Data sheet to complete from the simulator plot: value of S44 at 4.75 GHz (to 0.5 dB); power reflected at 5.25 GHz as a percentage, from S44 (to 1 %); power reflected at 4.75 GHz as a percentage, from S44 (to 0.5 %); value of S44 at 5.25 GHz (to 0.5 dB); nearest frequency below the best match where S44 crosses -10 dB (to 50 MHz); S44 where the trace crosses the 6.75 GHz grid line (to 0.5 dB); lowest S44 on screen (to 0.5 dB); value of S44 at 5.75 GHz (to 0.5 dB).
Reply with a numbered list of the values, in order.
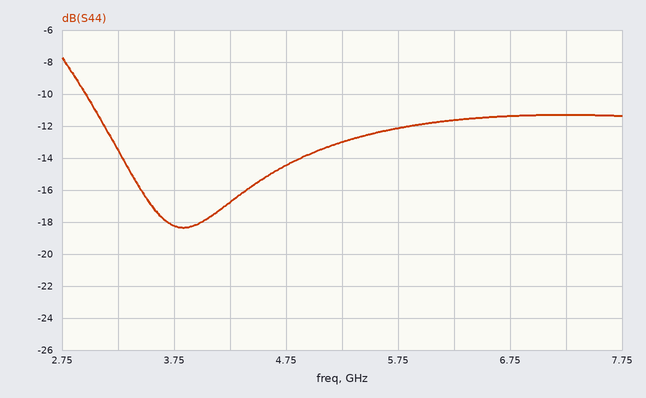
1. -14.5 dB
2. 5 %
3. 3.5 %
4. -13.0 dB
5. 2.95 GHz
6. -11.5 dB
7. -18.5 dB
8. -12.0 dB
